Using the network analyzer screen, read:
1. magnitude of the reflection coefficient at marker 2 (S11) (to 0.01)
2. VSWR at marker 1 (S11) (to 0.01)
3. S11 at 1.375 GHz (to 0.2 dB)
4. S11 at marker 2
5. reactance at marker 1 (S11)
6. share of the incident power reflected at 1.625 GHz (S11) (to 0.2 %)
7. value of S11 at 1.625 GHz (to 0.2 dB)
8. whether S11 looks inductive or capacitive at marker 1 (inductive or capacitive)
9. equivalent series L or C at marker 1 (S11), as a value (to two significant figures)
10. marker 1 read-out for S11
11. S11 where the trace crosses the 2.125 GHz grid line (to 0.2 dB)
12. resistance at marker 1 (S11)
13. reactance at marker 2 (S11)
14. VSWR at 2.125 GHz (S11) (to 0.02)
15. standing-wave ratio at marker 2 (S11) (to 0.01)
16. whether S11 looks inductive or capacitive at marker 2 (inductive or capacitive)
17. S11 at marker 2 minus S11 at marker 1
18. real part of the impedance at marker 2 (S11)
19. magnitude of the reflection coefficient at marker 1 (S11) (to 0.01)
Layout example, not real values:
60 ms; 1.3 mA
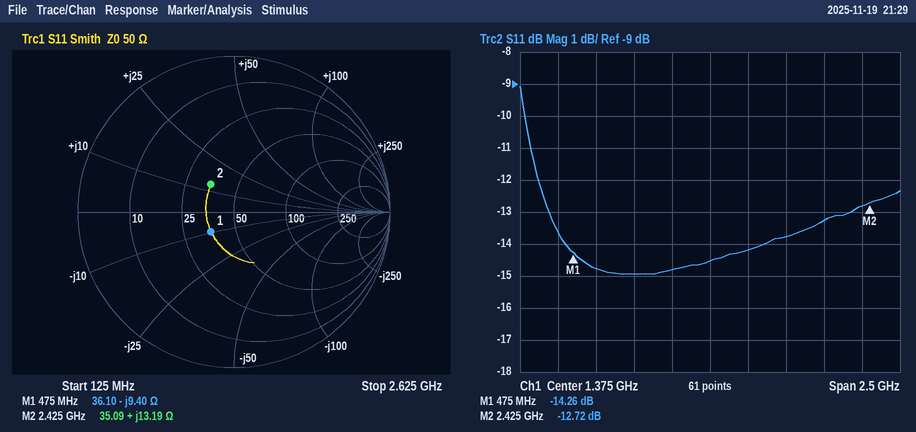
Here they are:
0.23; 1.48; -14.6 dB; -12.72 dB; -9.40 Ω; 3.8 %; -14.2 dB; capacitive; 36 pF; -14.26 dB; -13.2 dB; 36.10 Ω; +13.19 Ω; 1.56; 1.60; inductive; 1.54 dB; 35.09 Ω; 0.19
